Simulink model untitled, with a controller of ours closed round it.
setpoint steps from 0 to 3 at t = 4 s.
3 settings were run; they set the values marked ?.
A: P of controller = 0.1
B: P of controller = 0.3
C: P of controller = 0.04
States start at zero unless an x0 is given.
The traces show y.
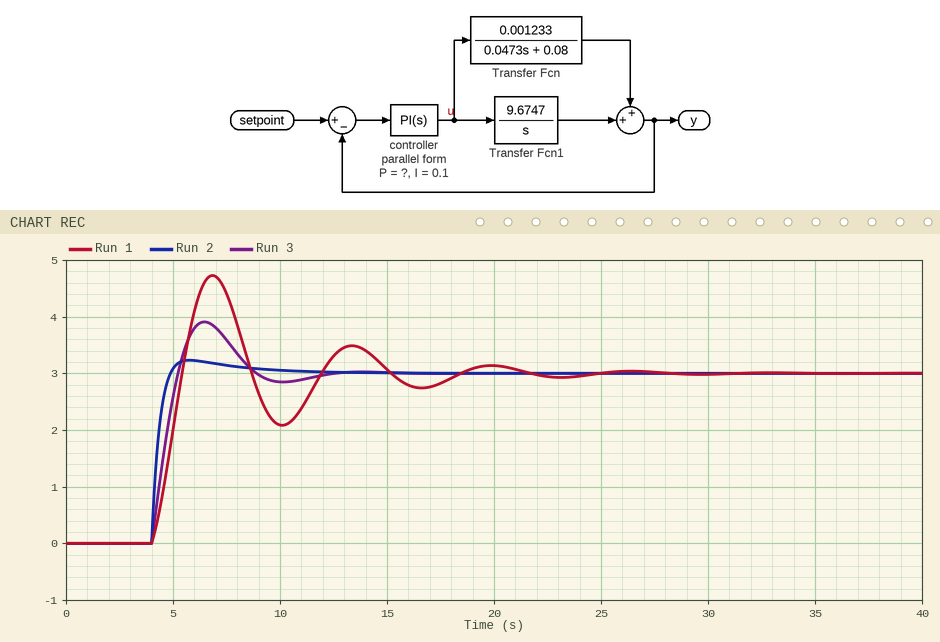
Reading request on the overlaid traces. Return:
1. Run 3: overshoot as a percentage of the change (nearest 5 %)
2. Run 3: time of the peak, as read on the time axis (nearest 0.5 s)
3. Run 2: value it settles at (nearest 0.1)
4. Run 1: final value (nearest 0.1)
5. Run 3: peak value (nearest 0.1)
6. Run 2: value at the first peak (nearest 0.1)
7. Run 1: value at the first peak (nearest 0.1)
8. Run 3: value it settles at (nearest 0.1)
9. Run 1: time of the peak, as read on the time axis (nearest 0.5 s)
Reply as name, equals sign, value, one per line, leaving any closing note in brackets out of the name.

Run 3: overshoot as a percentage of the change = 30 %
Run 3: time of the peak, as read on the time axis = 6.5 s
Run 2: value it settles at = 3.0
Run 1: final value = 3.0
Run 3: peak value = 3.9
Run 2: value at the first peak = 3.2
Run 1: value at the first peak = 4.7
Run 3: value it settles at = 3.0
Run 1: time of the peak, as read on the time axis = 7.0 s
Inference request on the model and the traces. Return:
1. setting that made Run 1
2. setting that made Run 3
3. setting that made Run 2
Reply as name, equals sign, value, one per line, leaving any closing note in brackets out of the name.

setting that made Run 1 = C
setting that made Run 3 = A
setting that made Run 2 = B
